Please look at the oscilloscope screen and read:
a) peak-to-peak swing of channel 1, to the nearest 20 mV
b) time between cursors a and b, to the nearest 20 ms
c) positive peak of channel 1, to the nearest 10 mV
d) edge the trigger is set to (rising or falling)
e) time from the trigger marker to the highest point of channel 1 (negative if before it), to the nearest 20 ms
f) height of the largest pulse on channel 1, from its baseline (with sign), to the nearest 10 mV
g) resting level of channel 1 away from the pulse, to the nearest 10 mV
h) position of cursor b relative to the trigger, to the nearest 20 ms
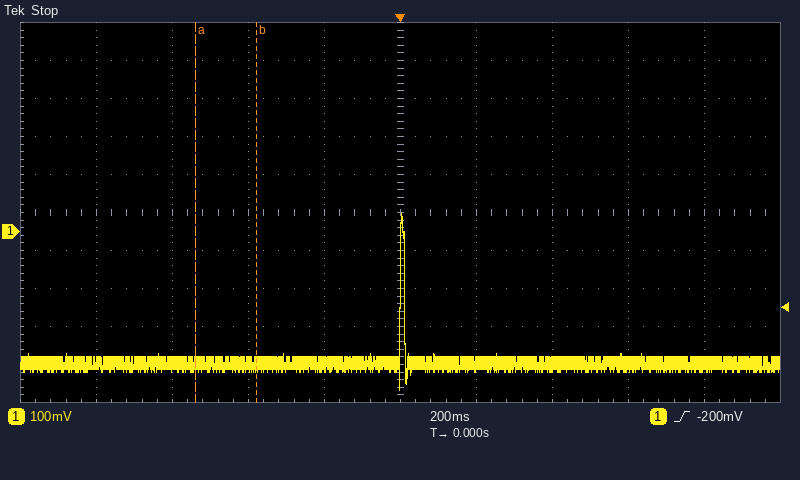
460 mV
160 ms
50 mV
rising
0 ms
+390 mV
-340 mV
-380 ms
